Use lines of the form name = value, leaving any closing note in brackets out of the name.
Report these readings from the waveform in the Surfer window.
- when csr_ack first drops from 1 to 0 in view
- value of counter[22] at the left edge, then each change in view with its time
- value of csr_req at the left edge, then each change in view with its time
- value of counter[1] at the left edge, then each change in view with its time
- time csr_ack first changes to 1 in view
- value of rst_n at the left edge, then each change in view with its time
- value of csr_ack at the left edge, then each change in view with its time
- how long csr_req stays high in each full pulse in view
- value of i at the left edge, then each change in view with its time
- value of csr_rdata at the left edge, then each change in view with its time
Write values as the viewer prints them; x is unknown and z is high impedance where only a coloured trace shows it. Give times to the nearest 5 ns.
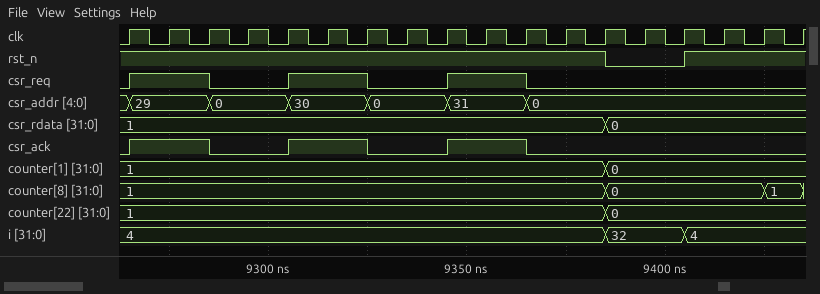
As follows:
when csr_ack first drops from 1 to 0 in view = 9285 ns
value of counter[22] at the left edge, then each change in view with its time = 1, 0 at 9385 ns
value of csr_req at the left edge, then each change in view with its time = 0, 1 at 9265 ns, 0 at 9285 ns, 1 at 9305 ns, 0 at 9325 ns, 1 at 9345 ns, 0 at 9365 ns
value of counter[1] at the left edge, then each change in view with its time = 1, 0 at 9385 ns
time csr_ack first changes to 1 in view = 9265 ns
value of rst_n at the left edge, then each change in view with its time = 1, 0 at 9385 ns, 1 at 9405 ns
value of csr_ack at the left edge, then each change in view with its time = 0, 1 at 9265 ns, 0 at 9285 ns, 1 at 9305 ns, 0 at 9325 ns, 1 at 9345 ns, 0 at 9365 ns
how long csr_req stays high in each full pulse in view = 20 ns, 20 ns, 20 ns
value of i at the left edge, then each change in view with its time = 4, 32 at 9385 ns, 4 at 9405 ns
value of csr_rdata at the left edge, then each change in view with its time = 1, 0 at 9385 ns
